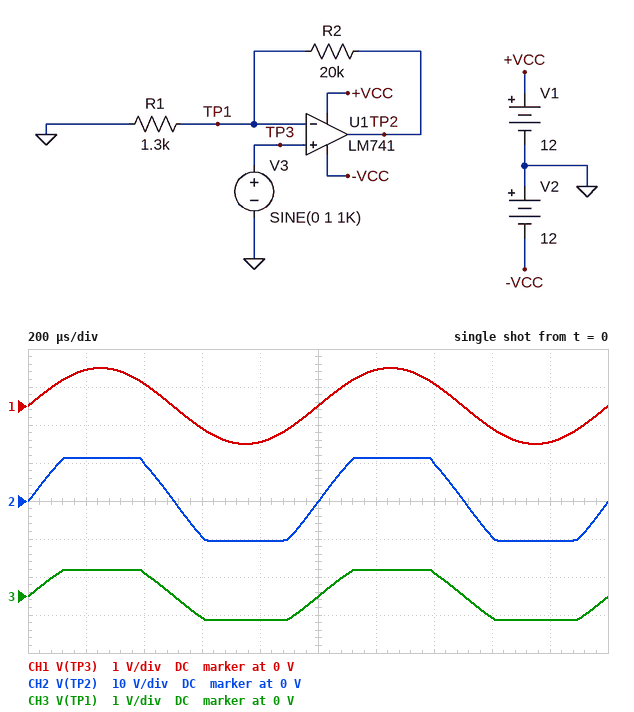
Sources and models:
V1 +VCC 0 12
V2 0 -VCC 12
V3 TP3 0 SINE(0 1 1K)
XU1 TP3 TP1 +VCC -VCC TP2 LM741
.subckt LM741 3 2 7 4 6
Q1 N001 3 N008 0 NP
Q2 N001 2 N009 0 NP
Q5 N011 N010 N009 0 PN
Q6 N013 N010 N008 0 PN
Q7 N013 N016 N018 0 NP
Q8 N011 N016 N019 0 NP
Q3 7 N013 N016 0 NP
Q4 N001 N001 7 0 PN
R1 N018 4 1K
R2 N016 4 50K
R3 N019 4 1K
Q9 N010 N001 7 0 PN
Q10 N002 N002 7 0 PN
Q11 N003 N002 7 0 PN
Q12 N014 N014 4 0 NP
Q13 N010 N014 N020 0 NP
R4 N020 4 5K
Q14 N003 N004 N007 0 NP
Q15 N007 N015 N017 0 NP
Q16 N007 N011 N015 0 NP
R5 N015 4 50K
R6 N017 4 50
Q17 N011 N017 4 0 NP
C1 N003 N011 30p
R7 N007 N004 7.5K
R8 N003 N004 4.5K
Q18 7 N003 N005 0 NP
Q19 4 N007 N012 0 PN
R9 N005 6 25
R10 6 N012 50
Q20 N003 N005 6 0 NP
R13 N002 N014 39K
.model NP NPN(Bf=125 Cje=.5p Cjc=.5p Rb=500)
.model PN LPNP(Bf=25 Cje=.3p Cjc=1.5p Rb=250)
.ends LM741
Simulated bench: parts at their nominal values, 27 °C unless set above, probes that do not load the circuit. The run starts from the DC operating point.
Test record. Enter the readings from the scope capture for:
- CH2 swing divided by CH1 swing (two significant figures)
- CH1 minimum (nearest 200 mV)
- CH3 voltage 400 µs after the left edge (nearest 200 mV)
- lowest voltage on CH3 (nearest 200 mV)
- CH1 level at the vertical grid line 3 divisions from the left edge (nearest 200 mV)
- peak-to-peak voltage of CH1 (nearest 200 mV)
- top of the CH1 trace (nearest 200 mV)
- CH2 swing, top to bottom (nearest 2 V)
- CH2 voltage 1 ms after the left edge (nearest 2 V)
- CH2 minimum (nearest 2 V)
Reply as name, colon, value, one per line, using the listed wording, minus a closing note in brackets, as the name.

CH2 swing divided by CH1 swing: 11
CH1 minimum: -1.0 V
CH3 voltage 400 µs after the left edge: 600 mV
lowest voltage on CH3: -600 mV
CH1 level at the vertical grid line 3 divisions from the left edge: -600 mV
peak-to-peak voltage of CH1: 2.0 V
top of the CH1 trace: 1.0 V
CH2 swing, top to bottom: 22 V
CH2 voltage 1 ms after the left edge: 0 V
CH2 minimum: -10 V
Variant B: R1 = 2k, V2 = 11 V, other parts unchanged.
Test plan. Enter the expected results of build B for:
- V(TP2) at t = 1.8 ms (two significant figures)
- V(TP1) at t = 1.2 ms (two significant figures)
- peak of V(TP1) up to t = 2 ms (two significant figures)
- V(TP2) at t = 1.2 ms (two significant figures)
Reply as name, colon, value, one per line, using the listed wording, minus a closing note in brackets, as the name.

V(TP2) at t = 1.8 ms: -9.4 V
V(TP1) at t = 1.2 ms: 950 mV
peak of V(TP1) up to t = 2 ms: 1.0 V
V(TP2) at t = 1.2 ms: 10 V
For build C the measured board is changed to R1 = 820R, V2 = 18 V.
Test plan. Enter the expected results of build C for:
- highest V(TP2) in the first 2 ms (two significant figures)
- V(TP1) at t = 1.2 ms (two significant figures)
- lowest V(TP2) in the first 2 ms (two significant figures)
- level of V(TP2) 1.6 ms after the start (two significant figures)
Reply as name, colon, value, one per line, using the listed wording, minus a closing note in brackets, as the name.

highest V(TP2) in the first 2 ms: 11 V
V(TP1) at t = 1.2 ms: 440 mV
lowest V(TP2) in the first 2 ms: -16 V
level of V(TP2) 1.6 ms after the start: -14 V
